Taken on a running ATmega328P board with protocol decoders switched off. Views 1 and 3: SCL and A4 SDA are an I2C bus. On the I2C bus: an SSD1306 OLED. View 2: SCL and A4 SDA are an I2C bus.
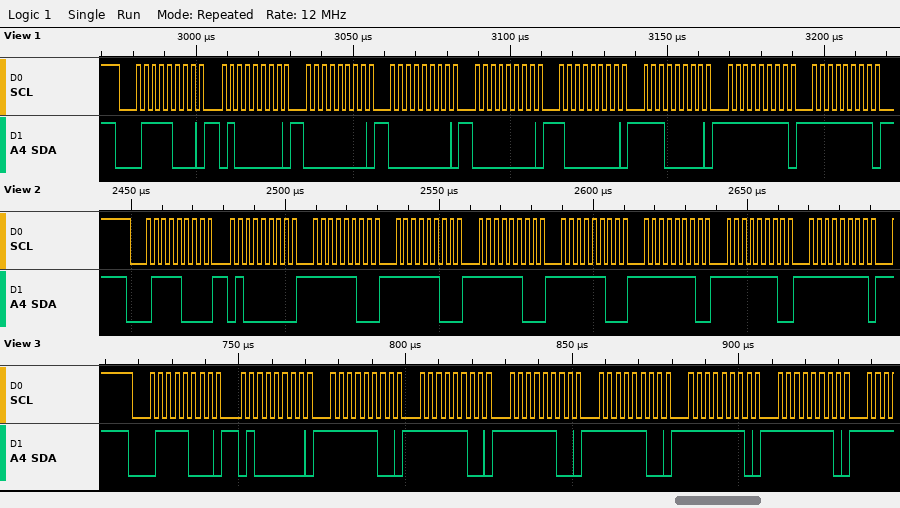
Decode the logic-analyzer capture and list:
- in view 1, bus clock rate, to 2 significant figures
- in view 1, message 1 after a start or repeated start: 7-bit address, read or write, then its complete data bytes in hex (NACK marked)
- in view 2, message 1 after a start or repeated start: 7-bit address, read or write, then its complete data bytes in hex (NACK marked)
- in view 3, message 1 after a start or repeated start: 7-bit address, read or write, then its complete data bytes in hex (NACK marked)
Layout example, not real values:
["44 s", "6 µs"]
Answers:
["400 kHz", "0x3C write: 40 00 00 00 80 E0 FF FF", "0x3C write: 40 FC FC FC FC FE FE FF", "0x3C write: 40 FC FC FC FC FE FE"]
